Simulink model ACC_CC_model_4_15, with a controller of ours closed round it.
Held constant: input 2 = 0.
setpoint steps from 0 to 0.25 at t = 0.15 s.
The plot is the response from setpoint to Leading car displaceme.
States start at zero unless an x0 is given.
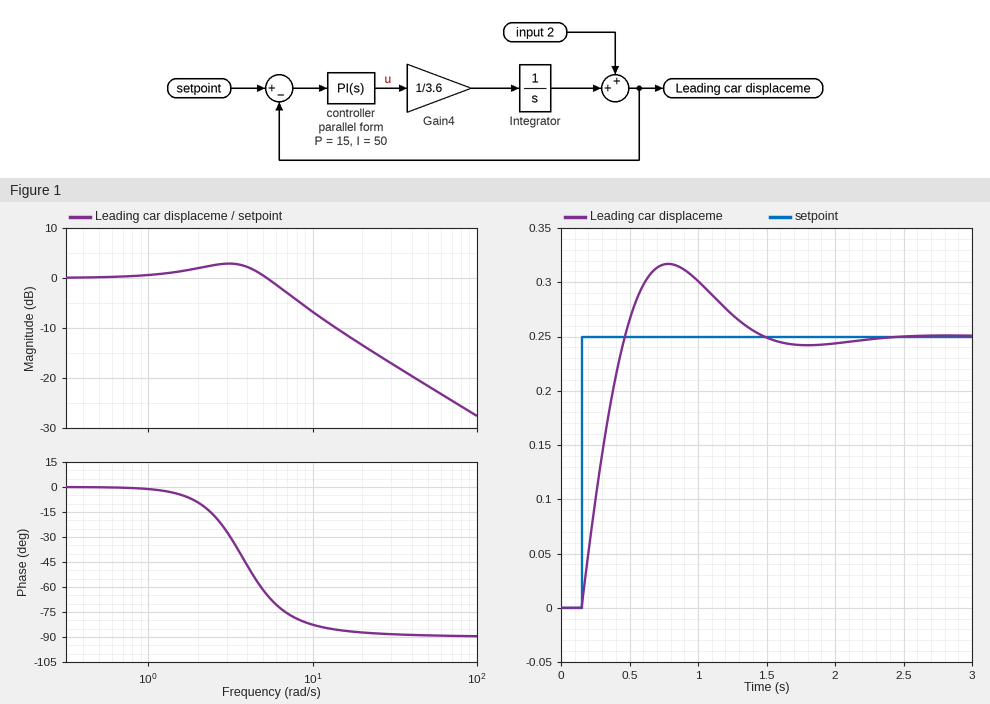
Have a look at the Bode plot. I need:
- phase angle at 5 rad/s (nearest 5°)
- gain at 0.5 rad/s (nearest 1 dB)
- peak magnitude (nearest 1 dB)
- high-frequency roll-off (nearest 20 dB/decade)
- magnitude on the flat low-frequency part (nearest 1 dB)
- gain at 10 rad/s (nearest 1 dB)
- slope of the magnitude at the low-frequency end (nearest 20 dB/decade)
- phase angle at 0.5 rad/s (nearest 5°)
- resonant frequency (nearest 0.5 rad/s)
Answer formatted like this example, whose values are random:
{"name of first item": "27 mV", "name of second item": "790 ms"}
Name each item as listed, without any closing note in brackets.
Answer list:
{"phase angle at 5 rad/s": "-60°", "gain at 0.5 rad/s": "0 dB", "peak magnitude": "3 dB", "high-frequency roll-off": "-20 dB/decade", "magnitude on the flat low-frequency part": "0 dB", "gain at 10 rad/s": "-7 dB", "slope of the magnitude at the low-frequency end": "0 dB/decade", "phase angle at 0.5 rad/s": "0°", "resonant frequency": "3.0 rad/s"}
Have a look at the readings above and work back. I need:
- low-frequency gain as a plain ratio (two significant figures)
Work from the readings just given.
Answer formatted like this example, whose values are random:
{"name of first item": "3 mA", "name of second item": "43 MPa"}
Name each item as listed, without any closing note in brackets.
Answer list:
{"low-frequency gain as a plain ratio": "1.0"}
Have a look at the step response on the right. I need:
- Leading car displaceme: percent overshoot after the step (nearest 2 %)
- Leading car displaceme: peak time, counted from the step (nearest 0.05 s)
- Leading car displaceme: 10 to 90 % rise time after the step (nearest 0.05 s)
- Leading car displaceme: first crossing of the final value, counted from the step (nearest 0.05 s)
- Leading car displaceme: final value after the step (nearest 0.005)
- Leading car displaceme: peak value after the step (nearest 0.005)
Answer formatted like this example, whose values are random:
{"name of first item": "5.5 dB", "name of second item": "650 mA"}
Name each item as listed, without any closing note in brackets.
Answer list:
{"Leading car displaceme: percent overshoot after the step": "26 %", "Leading car displaceme: peak time, counted from the step": "0.65 s", "Leading car displaceme: 10 to 90 % rise time after the step": "0.25 s", "Leading car displaceme: first crossing of the final value, counted from the step": "0.30 s", "Leading car displaceme: final value after the step": "0.250", "Leading car displaceme: peak value after the step": "0.315"}
